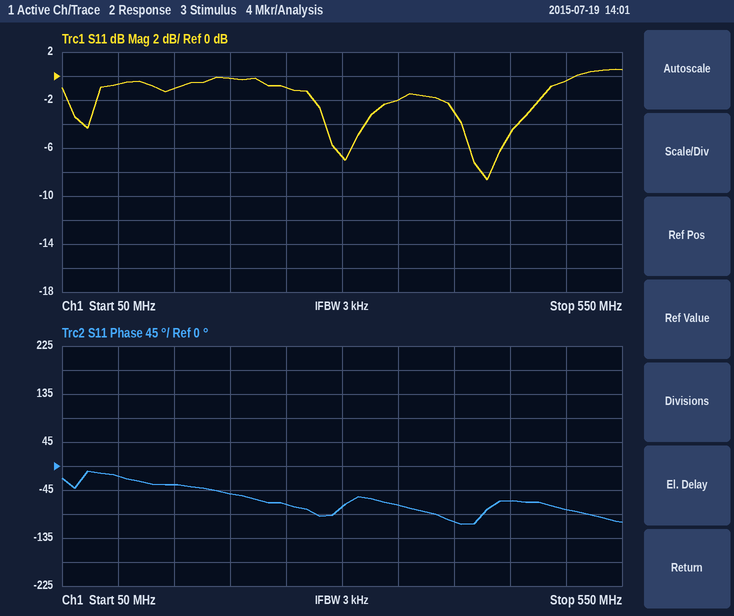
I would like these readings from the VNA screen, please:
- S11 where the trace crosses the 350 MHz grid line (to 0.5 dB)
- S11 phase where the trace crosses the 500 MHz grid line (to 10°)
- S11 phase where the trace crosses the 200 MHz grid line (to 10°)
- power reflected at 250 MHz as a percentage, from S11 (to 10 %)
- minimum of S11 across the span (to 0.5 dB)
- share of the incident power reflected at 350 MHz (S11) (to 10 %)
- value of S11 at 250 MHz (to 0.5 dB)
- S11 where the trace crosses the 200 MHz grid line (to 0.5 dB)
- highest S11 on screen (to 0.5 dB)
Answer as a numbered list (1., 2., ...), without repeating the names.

1. -2.0 dB
2. -80°
3. -50°
4. 80 %
5. -8.5 dB
6. 60 %
7. -1.0 dB
8. 0.0 dB
9. 0.5 dB
